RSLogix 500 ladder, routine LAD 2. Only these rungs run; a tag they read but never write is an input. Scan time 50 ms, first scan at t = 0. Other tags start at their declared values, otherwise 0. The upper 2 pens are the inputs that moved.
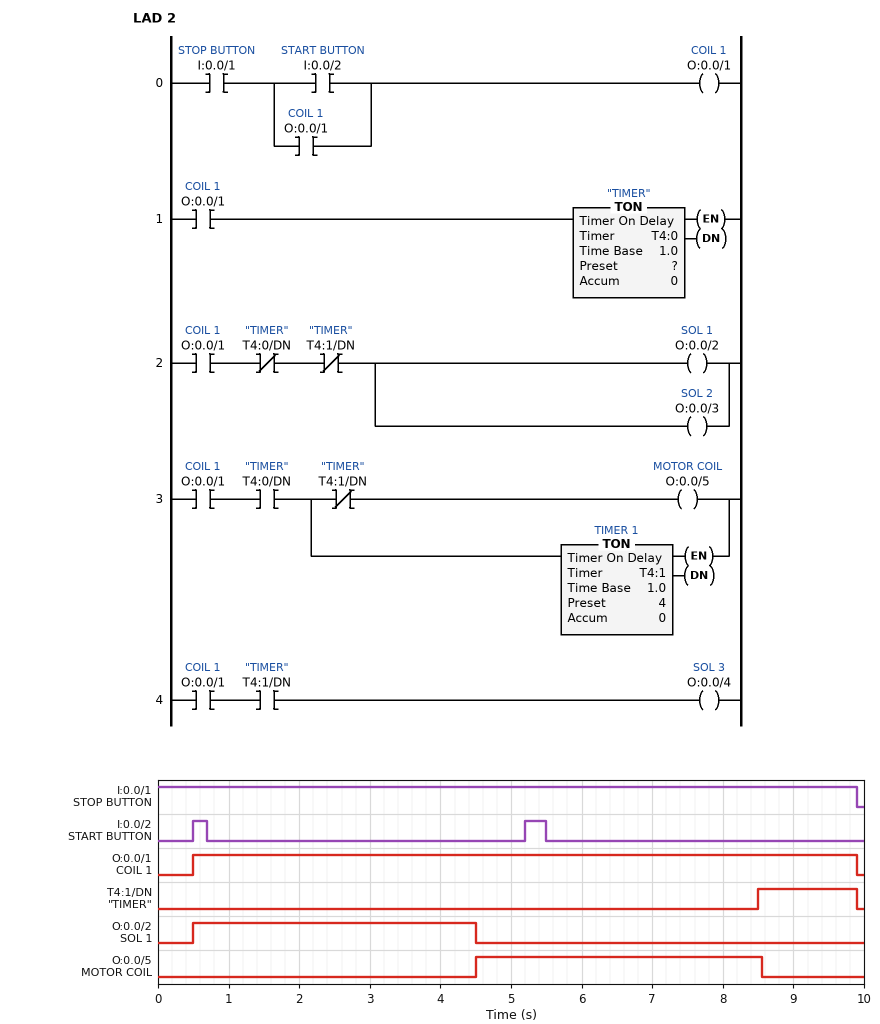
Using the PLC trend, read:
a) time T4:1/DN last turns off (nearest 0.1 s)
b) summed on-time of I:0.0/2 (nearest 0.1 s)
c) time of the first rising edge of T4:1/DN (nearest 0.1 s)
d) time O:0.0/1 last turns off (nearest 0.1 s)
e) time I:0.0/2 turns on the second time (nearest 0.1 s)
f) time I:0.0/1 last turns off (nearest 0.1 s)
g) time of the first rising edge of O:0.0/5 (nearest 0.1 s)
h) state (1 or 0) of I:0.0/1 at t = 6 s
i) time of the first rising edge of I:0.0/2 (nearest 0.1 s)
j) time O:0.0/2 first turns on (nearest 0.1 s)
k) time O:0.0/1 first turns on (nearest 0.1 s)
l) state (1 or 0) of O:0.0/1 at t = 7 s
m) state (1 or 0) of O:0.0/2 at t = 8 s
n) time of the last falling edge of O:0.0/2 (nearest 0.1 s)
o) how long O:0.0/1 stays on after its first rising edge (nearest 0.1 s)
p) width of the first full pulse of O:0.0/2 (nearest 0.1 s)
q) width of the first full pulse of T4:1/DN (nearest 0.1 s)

9.9 s
0.5 s
8.5 s
9.9 s
5.2 s
9.9 s
4.5 s
1
0.5 s
0.5 s
0.5 s
1
0
4.5 s
9.4 s
4.0 s
1.4 s
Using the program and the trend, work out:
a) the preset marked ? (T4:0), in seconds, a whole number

4 s
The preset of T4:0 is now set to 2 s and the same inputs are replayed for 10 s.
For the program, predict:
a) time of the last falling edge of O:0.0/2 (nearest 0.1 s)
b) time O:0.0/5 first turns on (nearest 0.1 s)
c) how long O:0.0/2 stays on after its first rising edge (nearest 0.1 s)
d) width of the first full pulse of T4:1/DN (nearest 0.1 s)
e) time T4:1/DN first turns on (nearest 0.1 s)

2.5 s
2.5 s
2.0 s
3.4 s
6.5 s
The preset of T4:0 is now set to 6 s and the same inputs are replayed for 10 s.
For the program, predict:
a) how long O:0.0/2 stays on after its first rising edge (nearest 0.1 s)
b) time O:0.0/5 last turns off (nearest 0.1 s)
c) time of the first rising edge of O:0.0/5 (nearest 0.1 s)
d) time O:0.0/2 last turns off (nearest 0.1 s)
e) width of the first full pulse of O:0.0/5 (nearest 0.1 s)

6.0 s
9.9 s
6.5 s
6.5 s
3.4 s
